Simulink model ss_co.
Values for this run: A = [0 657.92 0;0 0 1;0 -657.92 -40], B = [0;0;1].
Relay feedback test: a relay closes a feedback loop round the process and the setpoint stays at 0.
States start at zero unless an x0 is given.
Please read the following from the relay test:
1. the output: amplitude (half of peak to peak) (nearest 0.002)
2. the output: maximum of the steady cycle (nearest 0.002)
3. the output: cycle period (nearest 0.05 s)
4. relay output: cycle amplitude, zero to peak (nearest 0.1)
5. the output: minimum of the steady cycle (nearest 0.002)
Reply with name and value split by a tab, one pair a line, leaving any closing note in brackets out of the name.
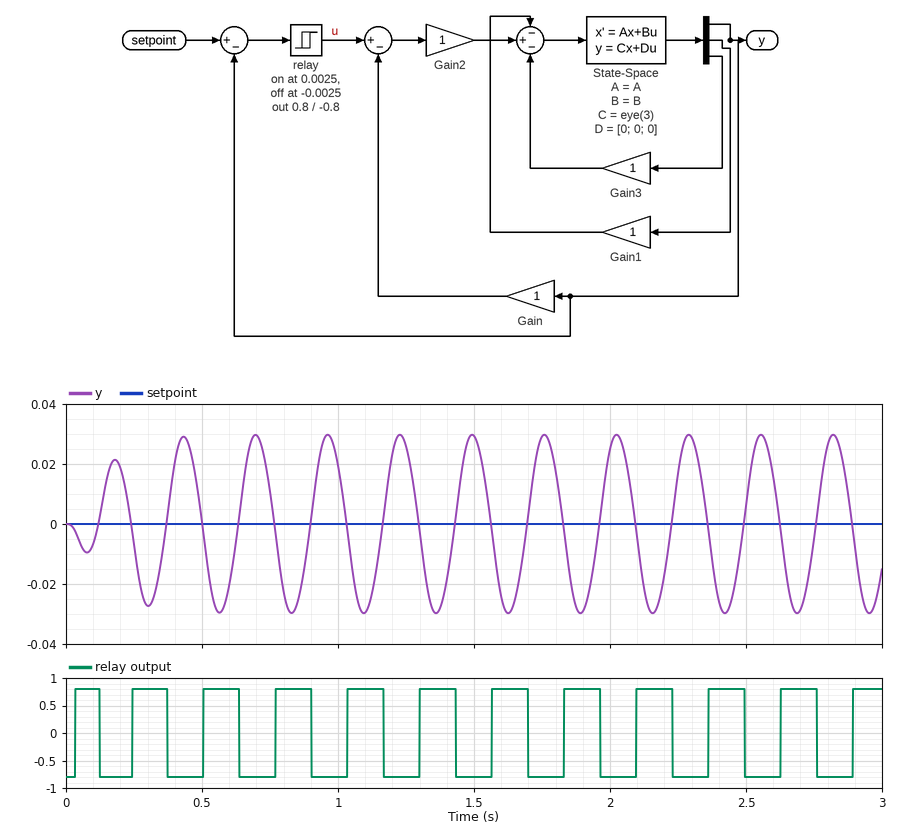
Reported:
the output: amplitude (half of peak to peak)	0.030
the output: maximum of the steady cycle	0.030
the output: cycle period	0.25 s
relay output: cycle amplitude, zero to peak	0.8
the output: minimum of the steady cycle	-0.030
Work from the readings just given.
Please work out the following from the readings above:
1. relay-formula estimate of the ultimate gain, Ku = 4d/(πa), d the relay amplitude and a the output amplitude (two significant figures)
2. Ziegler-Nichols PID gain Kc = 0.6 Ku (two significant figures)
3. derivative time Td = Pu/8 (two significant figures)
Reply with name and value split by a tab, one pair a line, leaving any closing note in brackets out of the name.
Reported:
relay-formula estimate of the ultimate gain, Ku = 4d/(πa), d the relay amplitude and a the output amplitude	34
Ziegler-Nichols PID gain Kc = 0.6 Ku	20
derivative time Td = Pu/8	0.031 s
